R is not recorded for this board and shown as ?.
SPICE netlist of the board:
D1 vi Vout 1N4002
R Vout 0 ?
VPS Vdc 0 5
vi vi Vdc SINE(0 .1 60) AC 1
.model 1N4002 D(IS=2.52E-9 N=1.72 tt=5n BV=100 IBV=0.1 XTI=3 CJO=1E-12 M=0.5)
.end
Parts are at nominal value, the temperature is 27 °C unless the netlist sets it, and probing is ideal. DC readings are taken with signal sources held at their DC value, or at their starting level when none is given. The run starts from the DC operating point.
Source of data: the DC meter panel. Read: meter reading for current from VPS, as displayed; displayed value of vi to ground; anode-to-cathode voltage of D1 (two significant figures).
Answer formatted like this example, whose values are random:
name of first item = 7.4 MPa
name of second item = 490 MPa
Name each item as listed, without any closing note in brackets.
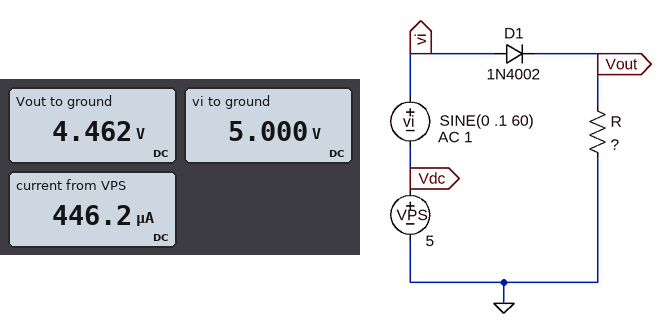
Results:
meter reading for current from VPS, as displayed = 446.2 µA
displayed value of vi to ground = 5.000 V
anode-to-cathode voltage of D1 = 540 mV
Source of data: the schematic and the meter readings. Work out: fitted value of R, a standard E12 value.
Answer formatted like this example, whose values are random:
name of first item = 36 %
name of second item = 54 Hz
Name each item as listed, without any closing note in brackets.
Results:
fitted value of R, a standard E12 value = 10 kΩ
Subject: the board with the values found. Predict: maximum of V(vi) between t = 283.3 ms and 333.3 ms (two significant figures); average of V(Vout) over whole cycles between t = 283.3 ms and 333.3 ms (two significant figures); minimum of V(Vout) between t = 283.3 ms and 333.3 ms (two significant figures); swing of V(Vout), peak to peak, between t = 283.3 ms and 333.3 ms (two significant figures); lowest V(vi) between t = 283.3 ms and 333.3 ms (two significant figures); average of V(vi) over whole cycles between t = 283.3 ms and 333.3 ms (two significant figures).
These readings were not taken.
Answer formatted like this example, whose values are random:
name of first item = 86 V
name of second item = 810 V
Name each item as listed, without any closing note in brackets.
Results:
maximum of V(vi) between t = 283.3 ms and 333.3 ms = 5.1 V
average of V(Vout) over whole cycles between t = 283.3 ms and 333.3 ms = 4.5 V
minimum of V(Vout) between t = 283.3 ms and 333.3 ms = 4.4 V
swing of V(Vout), peak to peak, between t = 283.3 ms and 333.3 ms = 200 mV
lowest V(vi) between t = 283.3 ms and 333.3 ms = 4.9 V
average of V(vi) over whole cycles between t = 283.3 ms and 333.3 ms = 5.0 V
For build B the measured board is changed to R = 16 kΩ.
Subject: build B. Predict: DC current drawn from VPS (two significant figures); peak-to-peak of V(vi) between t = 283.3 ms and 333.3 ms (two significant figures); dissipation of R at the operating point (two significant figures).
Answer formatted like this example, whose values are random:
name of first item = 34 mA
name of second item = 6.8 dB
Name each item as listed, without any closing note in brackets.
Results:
DC current drawn from VPS = 280 µA
peak-to-peak of V(vi) between t = 283.3 ms and 333.3 ms = 200 mV
dissipation of R at the operating point = 1.3 mW
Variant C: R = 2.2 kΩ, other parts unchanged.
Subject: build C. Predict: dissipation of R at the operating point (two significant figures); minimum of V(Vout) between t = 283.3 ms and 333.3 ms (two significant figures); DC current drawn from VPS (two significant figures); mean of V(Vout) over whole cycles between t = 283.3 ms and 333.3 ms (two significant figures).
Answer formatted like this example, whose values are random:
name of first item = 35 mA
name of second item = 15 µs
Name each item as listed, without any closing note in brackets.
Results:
dissipation of R at the operating point = 8.8 mW
minimum of V(Vout) between t = 283.3 ms and 333.3 ms = 4.3 V
DC current drawn from VPS = 2.0 mA
mean of V(Vout) over whole cycles between t = 283.3 ms and 333.3 ms = 4.4 V
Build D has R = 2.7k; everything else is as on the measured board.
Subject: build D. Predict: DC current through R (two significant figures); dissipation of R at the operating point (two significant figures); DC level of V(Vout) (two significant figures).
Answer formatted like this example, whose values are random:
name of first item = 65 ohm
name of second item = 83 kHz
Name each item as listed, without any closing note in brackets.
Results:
DC current through R = 1.6 mA
dissipation of R at the operating point = 7.2 mW
DC level of V(Vout) = 4.4 V
